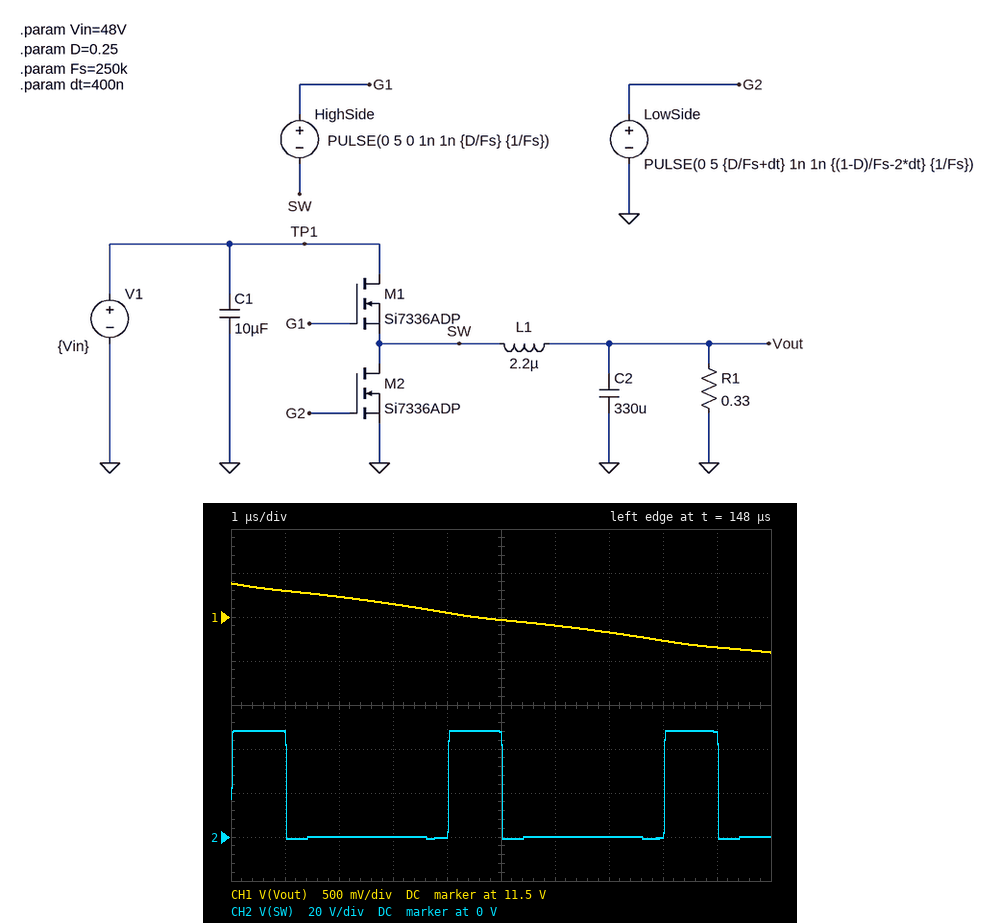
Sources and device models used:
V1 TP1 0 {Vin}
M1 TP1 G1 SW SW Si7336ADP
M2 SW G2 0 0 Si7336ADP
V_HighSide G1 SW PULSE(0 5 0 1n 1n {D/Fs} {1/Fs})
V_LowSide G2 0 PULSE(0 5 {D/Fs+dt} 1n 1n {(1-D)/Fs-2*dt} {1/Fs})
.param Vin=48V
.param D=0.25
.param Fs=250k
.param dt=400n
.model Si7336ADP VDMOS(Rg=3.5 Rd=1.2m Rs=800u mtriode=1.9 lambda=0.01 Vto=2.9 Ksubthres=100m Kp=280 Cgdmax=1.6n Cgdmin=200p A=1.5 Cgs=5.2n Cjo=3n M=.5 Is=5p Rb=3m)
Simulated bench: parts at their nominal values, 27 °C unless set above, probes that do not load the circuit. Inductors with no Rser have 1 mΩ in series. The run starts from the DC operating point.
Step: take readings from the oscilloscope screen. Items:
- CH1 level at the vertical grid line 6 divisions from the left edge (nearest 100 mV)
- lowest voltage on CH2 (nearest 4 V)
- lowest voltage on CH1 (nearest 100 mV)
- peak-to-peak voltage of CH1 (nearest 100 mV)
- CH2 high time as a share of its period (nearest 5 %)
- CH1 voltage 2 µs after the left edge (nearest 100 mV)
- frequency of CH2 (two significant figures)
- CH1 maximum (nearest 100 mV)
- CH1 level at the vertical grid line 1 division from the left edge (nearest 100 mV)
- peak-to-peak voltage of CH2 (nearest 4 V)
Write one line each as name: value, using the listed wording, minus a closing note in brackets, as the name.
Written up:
CH1 level at the vertical grid line 6 divisions from the left edge: 11.4 V
lowest voltage on CH2: 0 V
lowest voltage on CH1: 11.1 V
peak-to-peak voltage of CH1: 800 mV
CH2 high time as a share of its period: 25 %
CH1 voltage 2 µs after the left edge: 11.7 V
frequency of CH2: 250 kHz
CH1 maximum: 11.9 V
CH1 level at the vertical grid line 1 division from the left edge: 11.8 V
peak-to-peak voltage of CH2: 48 V
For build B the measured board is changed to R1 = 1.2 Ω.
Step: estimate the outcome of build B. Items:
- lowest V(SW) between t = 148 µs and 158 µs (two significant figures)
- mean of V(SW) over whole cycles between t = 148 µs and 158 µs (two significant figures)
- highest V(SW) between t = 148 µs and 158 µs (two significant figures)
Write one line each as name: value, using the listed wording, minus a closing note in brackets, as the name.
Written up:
lowest V(SW) between t = 148 µs and 158 µs: -730 mV
mean of V(SW) over whole cycles between t = 148 µs and 158 µs: 17 V
highest V(SW) between t = 148 µs and 158 µs: 49 V
